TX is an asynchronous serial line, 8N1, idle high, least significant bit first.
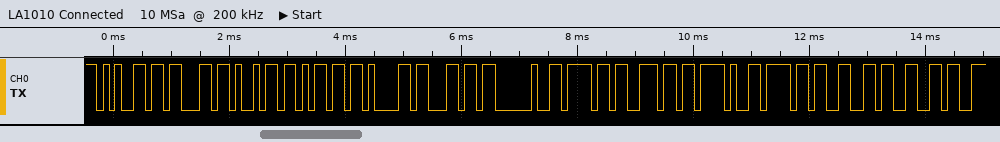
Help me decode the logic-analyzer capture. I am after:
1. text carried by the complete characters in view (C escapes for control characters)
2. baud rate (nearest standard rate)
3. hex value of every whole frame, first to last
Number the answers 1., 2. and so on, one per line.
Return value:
1. "ecimal on/off"
2. 9600 baud
3. 65 63 69 6D 61 6C 20 6F 6E 2F 6F 66 66
